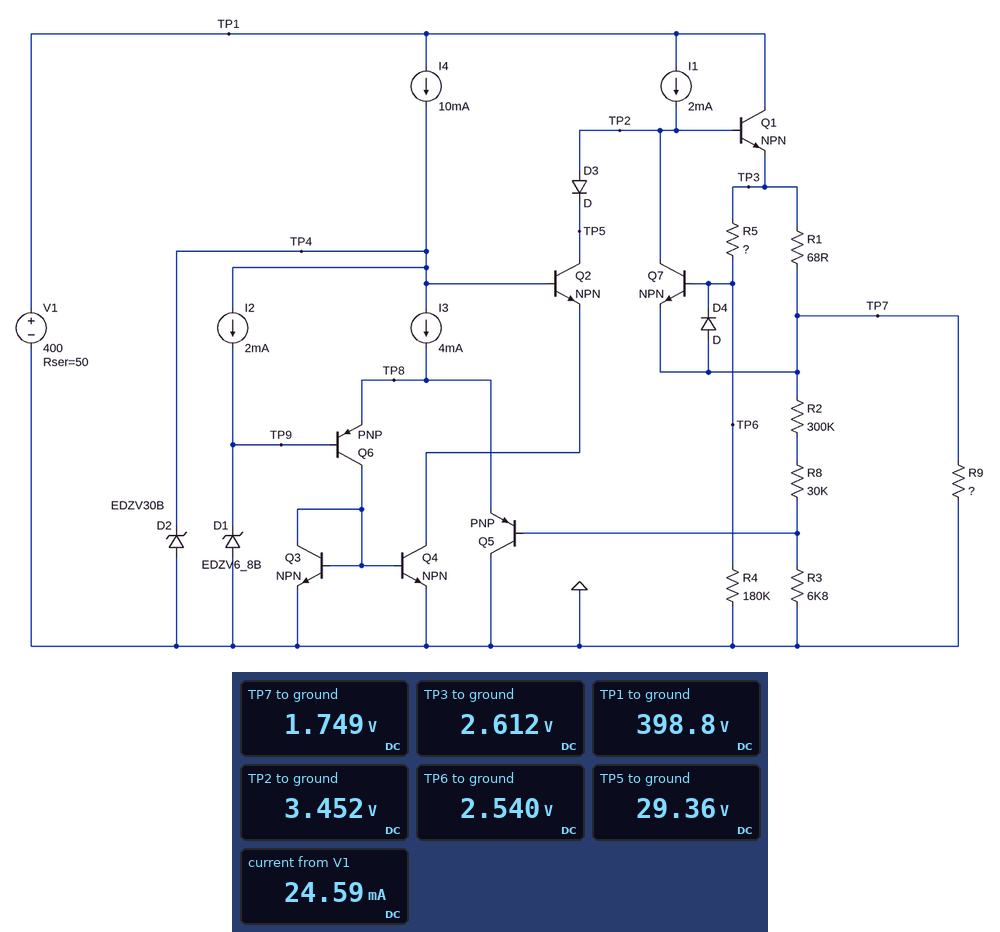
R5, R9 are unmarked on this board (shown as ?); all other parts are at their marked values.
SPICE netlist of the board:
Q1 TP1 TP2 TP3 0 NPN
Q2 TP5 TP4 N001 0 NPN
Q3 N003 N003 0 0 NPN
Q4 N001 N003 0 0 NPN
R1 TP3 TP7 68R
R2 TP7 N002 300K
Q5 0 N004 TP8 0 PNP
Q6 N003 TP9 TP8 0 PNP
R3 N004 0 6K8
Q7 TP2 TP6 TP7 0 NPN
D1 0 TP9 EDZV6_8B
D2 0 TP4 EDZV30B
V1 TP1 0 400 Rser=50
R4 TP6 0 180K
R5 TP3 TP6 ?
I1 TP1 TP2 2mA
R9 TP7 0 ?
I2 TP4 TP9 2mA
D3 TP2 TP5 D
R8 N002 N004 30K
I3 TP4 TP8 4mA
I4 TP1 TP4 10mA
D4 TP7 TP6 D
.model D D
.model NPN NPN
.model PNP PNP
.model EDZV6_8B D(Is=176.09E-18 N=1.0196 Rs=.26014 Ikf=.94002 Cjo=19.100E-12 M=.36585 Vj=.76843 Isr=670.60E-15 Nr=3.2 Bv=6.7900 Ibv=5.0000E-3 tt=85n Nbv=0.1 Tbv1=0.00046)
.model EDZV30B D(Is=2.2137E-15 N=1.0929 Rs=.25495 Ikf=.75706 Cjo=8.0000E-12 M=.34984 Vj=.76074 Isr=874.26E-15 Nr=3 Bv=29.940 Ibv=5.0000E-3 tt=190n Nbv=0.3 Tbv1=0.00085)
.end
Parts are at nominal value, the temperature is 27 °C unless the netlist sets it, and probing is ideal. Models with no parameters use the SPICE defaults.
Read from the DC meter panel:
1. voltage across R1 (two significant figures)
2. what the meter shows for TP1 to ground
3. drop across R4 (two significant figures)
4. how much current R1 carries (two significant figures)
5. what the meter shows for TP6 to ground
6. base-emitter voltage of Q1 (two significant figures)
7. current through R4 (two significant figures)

860 mV
398.8 V
2.5 V
13 mA
2.540 V
840 mV
14 µA
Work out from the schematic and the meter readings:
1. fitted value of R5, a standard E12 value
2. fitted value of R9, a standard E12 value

2.2 kΩ
120 Ω
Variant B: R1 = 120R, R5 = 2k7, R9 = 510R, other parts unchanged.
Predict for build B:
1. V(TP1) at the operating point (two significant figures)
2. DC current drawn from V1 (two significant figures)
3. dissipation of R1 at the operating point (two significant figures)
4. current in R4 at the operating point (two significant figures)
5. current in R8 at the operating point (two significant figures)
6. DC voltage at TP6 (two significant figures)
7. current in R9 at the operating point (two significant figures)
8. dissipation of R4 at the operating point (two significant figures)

400 V
20 mA
7.2 mW
32 µA
14 µA
5.7 V
9.7 mA
180 µW
